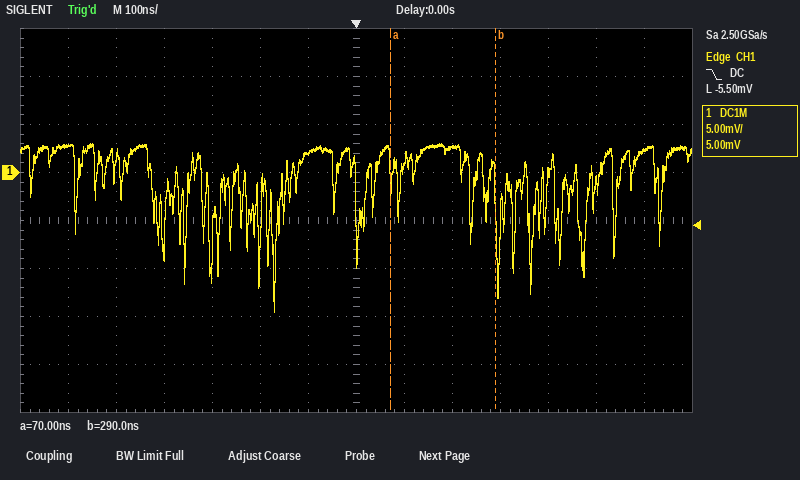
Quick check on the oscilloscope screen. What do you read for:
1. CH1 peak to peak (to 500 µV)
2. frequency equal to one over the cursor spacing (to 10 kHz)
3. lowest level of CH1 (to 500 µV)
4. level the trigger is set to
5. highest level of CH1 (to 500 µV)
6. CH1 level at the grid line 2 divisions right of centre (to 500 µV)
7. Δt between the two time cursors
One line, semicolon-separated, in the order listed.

17.5 mV; 4.55 MHz; -14.5 mV; -5.50 mV; 3.0 mV; 2.5 mV; 220 ns
